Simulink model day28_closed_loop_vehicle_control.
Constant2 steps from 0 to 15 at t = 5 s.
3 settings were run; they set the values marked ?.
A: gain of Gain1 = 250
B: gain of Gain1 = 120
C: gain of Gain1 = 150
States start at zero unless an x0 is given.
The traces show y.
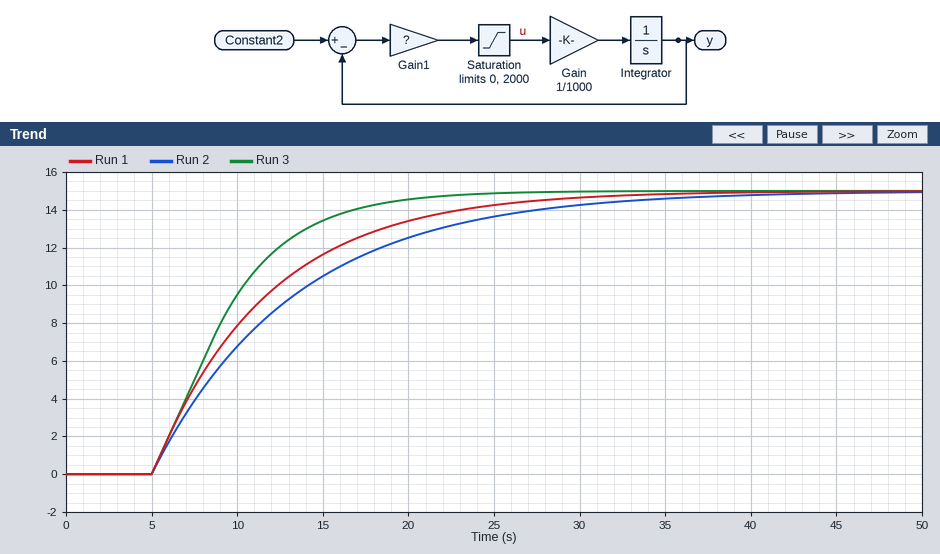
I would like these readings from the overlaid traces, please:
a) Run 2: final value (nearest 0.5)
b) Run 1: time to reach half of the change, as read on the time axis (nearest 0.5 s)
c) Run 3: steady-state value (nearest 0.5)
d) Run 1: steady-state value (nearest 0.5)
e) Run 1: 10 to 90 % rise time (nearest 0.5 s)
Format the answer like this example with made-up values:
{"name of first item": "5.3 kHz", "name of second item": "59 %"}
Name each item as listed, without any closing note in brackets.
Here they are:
{"Run 2: final value": "15.0", "Run 1: time to reach half of the change, as read on the time axis": "9.5 s", "Run 3: steady-state value": "15.0", "Run 1: steady-state value": "15.0", "Run 1: 10 to 90 % rise time": "14.5 s"}
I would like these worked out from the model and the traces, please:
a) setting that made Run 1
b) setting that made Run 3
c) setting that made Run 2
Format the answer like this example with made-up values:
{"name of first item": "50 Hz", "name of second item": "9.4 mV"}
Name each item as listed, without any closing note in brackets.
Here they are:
{"setting that made Run 1": "C", "setting that made Run 3": "A", "setting that made Run 2": "B"}
